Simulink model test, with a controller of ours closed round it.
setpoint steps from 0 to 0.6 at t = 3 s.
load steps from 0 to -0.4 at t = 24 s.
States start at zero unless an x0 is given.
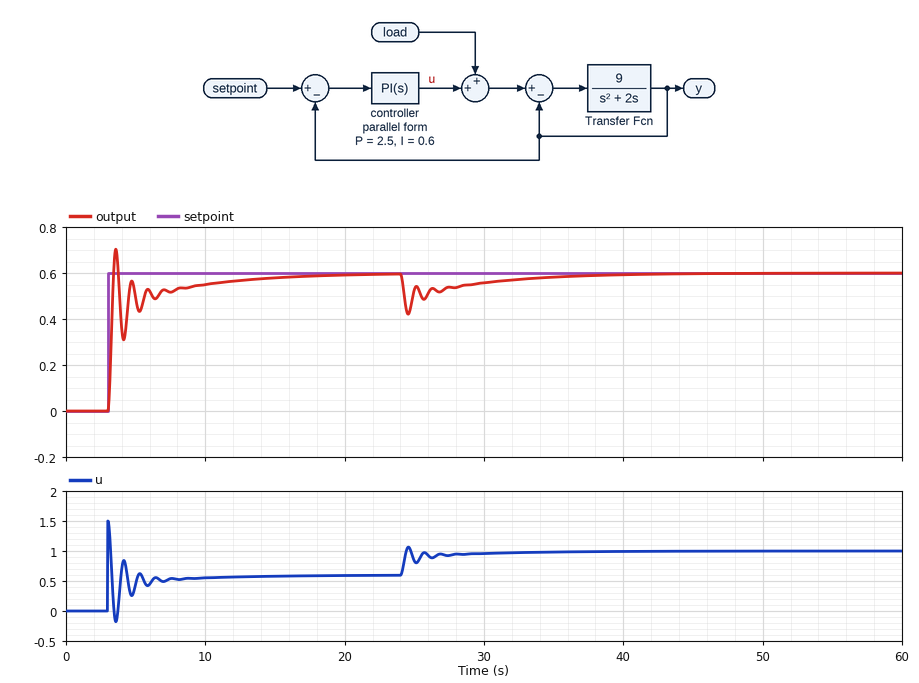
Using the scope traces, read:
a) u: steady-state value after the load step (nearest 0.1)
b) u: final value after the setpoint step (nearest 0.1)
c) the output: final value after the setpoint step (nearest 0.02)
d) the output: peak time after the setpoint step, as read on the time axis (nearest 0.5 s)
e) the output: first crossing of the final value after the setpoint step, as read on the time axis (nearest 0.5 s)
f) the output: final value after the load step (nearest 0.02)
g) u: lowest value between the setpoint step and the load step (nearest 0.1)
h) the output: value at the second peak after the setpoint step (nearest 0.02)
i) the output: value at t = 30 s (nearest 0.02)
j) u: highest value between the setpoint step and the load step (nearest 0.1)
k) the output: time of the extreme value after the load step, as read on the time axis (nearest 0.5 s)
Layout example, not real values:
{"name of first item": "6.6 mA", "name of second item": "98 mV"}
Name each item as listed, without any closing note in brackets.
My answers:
{"u: steady-state value after the load step": "1.0", "u: final value after the setpoint step": "0.6", "the output: final value after the setpoint step": "0.60", "the output: peak time after the setpoint step, as read on the time axis": "3.5 s", "the output: first crossing of the final value after the setpoint step, as read on the time axis": "3.5 s", "the output: final value after the load step": "0.60", "u: lowest value between the setpoint step and the load step": "-0.2", "the output: value at the second peak after the setpoint step": "0.56", "the output: value at t = 30 s": "0.56", "u: highest value between the setpoint step and the load step": "1.5", "the output: time of the extreme value after the load step, as read on the time axis": "24.5 s"}
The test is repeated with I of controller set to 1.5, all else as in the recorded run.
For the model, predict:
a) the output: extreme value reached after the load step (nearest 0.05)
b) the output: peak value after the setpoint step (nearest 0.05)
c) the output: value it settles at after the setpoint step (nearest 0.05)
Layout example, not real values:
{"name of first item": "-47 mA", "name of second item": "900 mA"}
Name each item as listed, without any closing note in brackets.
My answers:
{"the output: extreme value reached after the load step": "0.45", "the output: peak value after the setpoint step": "0.75", "the output: value it settles at after the setpoint step": "0.60"}
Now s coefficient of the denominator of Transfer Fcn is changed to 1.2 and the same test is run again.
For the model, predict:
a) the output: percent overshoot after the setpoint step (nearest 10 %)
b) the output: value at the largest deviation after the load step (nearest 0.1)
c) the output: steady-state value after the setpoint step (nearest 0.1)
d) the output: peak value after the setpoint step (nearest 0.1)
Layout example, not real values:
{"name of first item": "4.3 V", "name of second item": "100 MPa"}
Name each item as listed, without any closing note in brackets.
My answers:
{"the output: percent overshoot after the setpoint step": "30 %", "the output: value at the largest deviation after the load step": "0.4", "the output: steady-state value after the setpoint step": "0.6", "the output: peak value after the setpoint step": "0.8"}
